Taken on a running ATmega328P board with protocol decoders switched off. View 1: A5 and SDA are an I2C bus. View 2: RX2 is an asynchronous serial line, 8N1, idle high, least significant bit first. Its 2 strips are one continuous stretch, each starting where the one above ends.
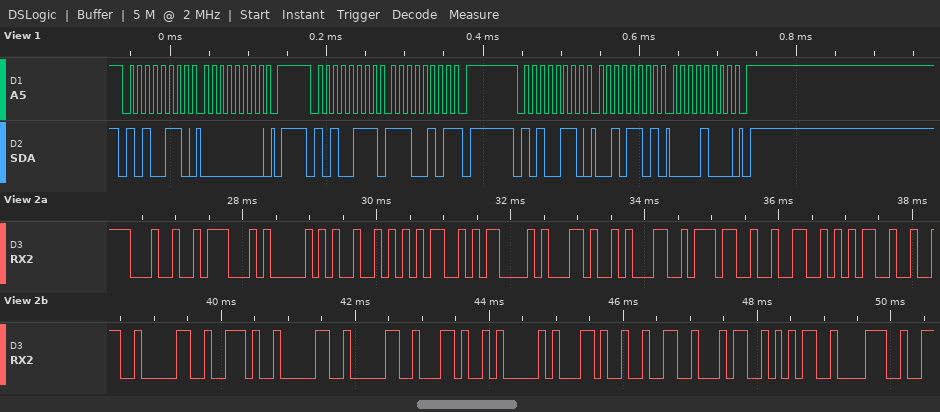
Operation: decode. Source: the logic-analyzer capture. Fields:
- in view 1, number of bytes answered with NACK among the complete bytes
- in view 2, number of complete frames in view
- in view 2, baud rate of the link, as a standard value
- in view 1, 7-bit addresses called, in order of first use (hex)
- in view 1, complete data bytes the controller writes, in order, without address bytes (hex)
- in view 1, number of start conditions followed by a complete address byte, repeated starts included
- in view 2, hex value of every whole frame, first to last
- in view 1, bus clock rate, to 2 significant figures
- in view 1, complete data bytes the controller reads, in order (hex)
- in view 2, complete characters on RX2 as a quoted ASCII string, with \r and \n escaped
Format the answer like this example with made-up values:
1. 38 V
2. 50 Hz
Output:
1. 1
2. 23
3. 9600 baud
4. 0x53
5. 00 2D 08
6. 3
7. 24 47 50 52 4D 43 2C 31 37 32 35 32 30 2E 30 30 2C 41 2C 32 34 35 38
8. 100 kHz
9. E5
10. "$GPRMC,172520.00,A,2458"
